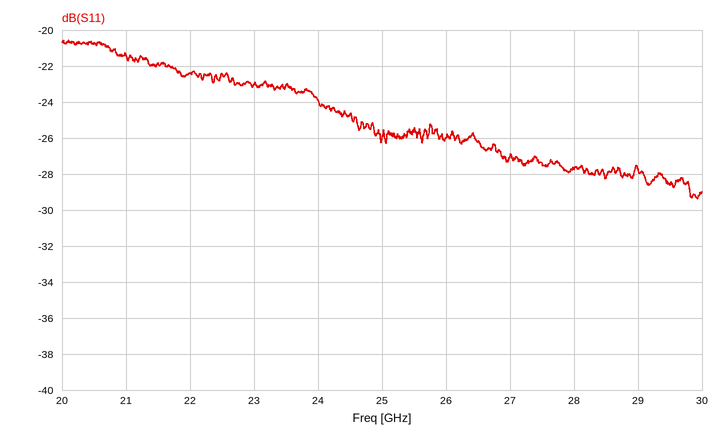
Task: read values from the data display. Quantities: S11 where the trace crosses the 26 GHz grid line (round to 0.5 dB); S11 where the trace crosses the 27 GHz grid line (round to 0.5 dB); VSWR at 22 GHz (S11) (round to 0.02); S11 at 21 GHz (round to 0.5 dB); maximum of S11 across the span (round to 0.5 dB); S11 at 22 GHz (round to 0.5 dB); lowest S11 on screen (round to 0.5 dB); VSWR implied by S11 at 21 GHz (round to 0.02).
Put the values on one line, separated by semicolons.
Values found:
-26.0 dB; -27.0 dB; 1.16; -21.5 dB; -20.5 dB; -22.5 dB; -29.5 dB; 1.18
